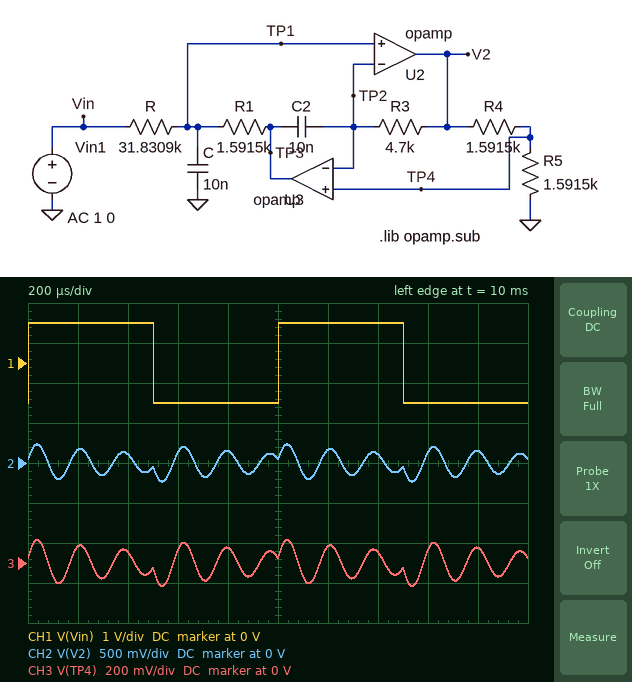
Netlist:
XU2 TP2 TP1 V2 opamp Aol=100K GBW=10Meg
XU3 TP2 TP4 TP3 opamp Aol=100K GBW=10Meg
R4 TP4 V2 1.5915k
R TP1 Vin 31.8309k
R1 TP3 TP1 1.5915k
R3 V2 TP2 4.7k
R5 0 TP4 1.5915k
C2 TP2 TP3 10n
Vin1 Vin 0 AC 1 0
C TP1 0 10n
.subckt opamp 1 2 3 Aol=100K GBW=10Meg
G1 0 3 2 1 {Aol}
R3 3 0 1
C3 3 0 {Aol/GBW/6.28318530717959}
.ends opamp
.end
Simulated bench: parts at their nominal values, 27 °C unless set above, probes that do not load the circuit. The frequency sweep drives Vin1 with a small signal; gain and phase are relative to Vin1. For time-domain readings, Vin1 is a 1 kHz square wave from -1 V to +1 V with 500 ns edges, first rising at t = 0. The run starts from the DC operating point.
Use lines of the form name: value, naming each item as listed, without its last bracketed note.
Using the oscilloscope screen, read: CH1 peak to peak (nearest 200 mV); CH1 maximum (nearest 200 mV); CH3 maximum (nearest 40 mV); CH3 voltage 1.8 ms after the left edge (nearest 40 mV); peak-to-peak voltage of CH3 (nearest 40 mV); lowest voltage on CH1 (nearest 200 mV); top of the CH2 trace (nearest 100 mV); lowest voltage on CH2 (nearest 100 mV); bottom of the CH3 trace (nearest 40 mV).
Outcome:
CH1 peak to peak: 2.0 V
CH1 maximum: 1.0 V
CH3 maximum: 120 mV
CH3 voltage 1.8 ms after the left edge: 80 mV
peak-to-peak voltage of CH3: 240 mV
lowest voltage on CH1: -1.0 V
top of the CH2 trace: 200 mV
lowest voltage on CH2: -200 mV
bottom of the CH3 trace: -120 mV
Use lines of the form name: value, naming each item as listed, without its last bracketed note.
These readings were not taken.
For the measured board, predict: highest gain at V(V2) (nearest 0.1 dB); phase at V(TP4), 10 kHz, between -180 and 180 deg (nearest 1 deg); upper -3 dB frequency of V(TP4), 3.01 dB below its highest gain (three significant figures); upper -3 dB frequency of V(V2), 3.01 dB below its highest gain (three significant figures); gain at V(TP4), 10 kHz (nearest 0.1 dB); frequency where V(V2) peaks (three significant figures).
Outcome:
highest gain at V(V2): 6.0 dB
phase at V(TP4), 10 kHz, between -180 and 180 deg: -86 deg
upper -3 dB frequency of V(TP4), 3.01 dB below its highest gain: 6.07 kHz
upper -3 dB frequency of V(V2), 3.01 dB below its highest gain: 6.07 kHz
gain at V(TP4), 10 kHz: -22.5 dB
frequency where V(V2) peaks: 5.81 kHz
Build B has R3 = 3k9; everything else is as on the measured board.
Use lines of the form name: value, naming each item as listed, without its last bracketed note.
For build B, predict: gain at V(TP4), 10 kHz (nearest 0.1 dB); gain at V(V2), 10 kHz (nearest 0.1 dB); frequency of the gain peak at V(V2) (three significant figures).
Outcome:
gain at V(TP4), 10 kHz: -21.5 dB
gain at V(V2), 10 kHz: -15.5 dB
frequency of the gain peak at V(V2): 6.38 kHz
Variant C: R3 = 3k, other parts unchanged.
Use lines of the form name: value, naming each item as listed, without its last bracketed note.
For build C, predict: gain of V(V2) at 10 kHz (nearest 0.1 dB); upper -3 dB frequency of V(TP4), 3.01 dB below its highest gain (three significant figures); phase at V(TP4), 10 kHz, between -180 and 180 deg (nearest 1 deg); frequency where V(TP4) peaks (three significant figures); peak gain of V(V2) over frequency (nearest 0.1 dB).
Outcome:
gain of V(V2) at 10 kHz: -13.5 dB
upper -3 dB frequency of V(TP4), 3.01 dB below its highest gain: 7.53 kHz
phase at V(TP4), 10 kHz, between -180 and 180 deg: -84 deg
frequency where V(TP4) peaks: 7.27 kHz
peak gain of V(V2) over frequency: 6.0 dB
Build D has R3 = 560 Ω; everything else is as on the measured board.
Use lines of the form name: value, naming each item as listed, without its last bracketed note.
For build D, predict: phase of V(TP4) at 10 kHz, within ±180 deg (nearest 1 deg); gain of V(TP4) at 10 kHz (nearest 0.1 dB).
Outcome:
phase of V(TP4) at 10 kHz, within ±180 deg: 88 deg
gain of V(TP4) at 10 kHz: -31.3 dB
